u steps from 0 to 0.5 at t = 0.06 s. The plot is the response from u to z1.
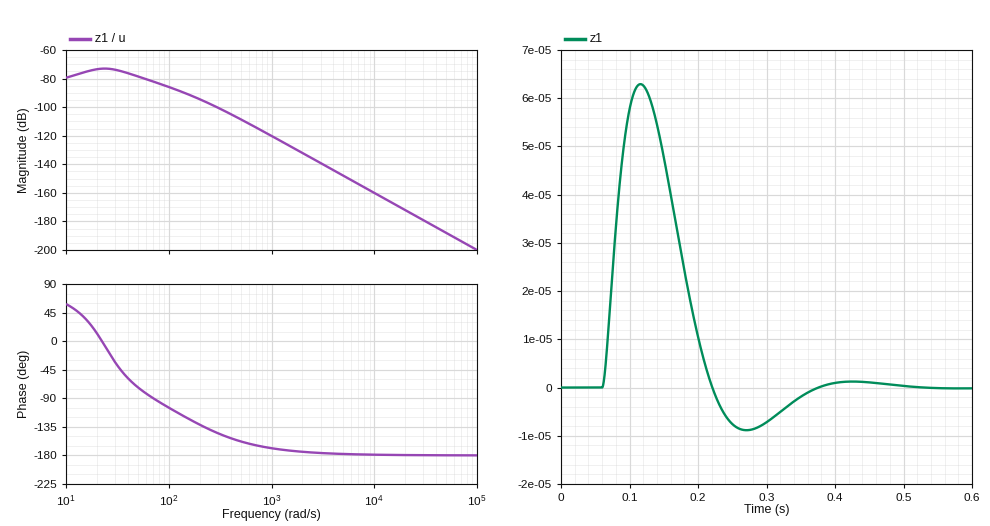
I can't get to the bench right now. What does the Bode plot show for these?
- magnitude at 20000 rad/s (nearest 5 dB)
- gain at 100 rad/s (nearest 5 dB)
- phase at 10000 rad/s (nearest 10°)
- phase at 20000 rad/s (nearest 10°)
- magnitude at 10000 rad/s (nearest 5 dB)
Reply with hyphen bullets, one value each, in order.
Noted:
- -170 dB
- -85 dB
- -180°
- -180°
- -160 dB
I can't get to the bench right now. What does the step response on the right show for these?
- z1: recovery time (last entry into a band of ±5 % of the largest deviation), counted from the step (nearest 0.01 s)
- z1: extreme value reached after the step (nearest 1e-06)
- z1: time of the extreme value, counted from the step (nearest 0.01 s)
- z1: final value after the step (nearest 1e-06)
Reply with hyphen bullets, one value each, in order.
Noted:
- 0.28 s
- 0.000063
- 0.06 s
- 0.000000
